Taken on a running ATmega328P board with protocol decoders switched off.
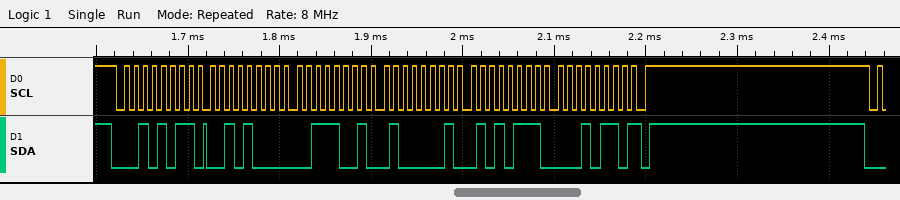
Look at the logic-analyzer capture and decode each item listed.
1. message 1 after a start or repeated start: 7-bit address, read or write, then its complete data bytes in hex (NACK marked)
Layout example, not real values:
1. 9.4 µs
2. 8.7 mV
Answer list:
1. 0x15 read: 28 39 41 57 16 NACK
